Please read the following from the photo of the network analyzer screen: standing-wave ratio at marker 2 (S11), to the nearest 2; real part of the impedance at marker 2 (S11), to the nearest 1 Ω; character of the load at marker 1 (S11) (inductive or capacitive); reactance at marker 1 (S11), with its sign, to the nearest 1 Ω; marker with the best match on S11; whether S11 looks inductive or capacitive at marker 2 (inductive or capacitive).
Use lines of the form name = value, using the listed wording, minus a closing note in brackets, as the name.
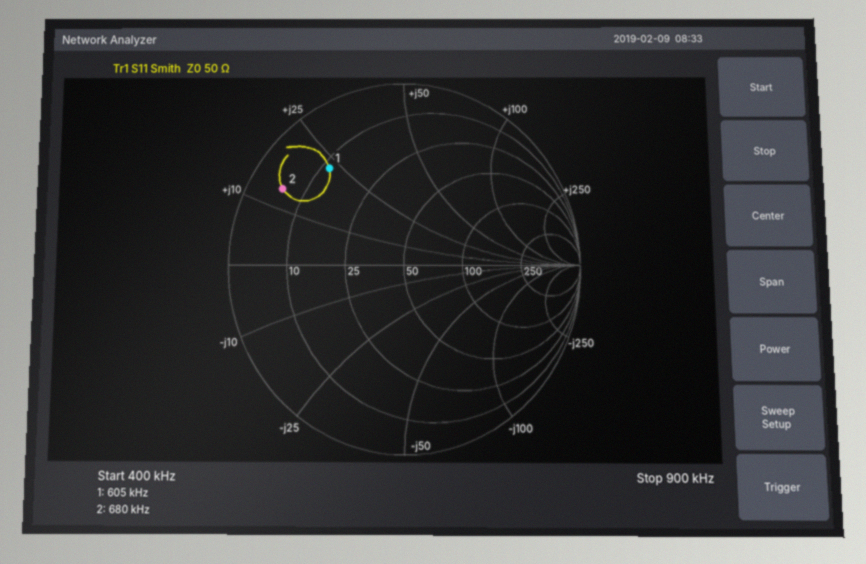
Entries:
standing-wave ratio at marker 2 (S11), to the nearest 2 = 10
real part of the impedance at marker 2 (S11), to the nearest 1 Ω = 6 Ω
character of the load at marker 1 (S11) = inductive
reactance at marker 1 (S11), with its sign, to the nearest 1 Ω = +23 Ω
marker with the best match on S11 = marker 1
whether S11 looks inductive or capacitive at marker 2 = inductive
